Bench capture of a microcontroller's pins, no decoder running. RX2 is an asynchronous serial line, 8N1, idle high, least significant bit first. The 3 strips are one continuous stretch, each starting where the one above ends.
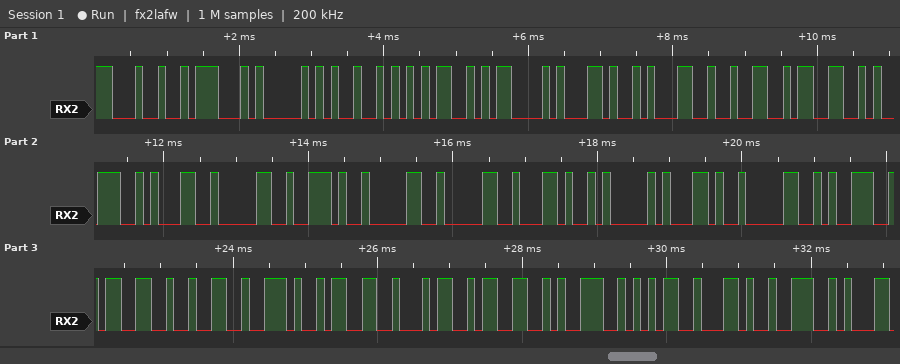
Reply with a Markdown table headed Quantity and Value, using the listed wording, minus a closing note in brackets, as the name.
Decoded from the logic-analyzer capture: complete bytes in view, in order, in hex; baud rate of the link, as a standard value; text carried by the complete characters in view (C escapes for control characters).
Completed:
| Quantity | Value |
|---|---|
| complete bytes in view, in order, in hex | 0x24 0x47 0x50 0x52 0x4D 0x43 0x2C 0x31 0x32 0x33 0x39 0x31 0x30 0x2E 0x30 0x30 0x2C 0x41 0x2C 0x30 0x39 0x33 0x32 0x2E 0x33 0x34 0x33 0x39 0x35 0x2C 0x4E |
| baud rate of the link, as a standard value | 9600 baud |
| text carried by the complete characters in view | "$GPRMC,123910.00,A,0932.34395,N" |
